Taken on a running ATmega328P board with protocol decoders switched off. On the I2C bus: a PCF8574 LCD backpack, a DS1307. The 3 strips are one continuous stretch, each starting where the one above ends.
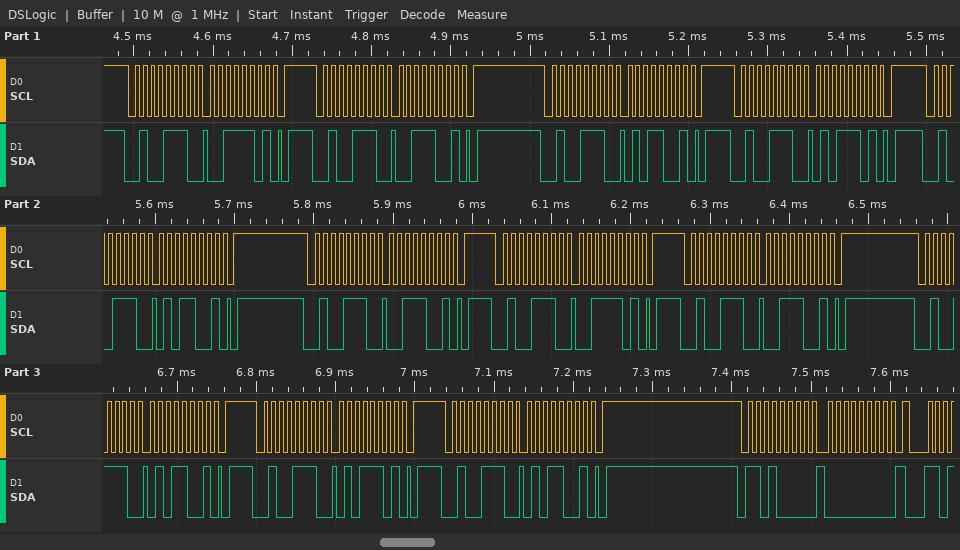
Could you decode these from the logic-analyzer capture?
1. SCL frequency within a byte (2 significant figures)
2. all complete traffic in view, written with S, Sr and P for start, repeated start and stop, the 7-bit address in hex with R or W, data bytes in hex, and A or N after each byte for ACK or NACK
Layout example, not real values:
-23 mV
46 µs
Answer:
100 kHz
S 27W A 3D A P S 27W A 39 A P S 27W A 59 A P S 27W A 5D A P S 27W A 59 A P S 27W A 39 A P S 27W A 3D A P S 27W A 39 A P S 27W A 59 A P S 27W A 5D A P S 27W A 59 A P S 68W A 00 A
